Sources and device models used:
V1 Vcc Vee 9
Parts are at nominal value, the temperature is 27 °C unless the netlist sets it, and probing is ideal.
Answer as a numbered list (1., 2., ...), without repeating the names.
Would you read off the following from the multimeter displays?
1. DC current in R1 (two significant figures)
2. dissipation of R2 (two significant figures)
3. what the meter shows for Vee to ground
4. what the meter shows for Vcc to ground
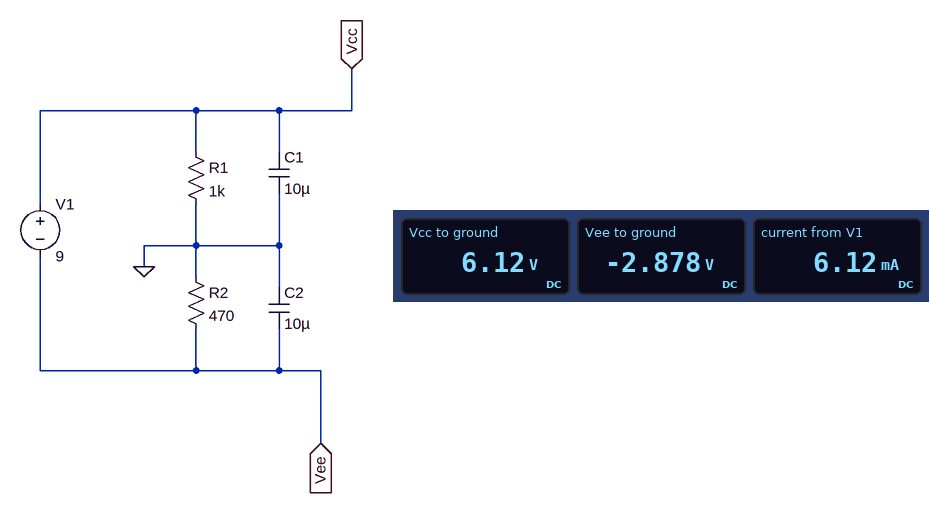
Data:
1. 6.1 mA
2. 18 mW
3. -2.878 V
4. 6.12 V
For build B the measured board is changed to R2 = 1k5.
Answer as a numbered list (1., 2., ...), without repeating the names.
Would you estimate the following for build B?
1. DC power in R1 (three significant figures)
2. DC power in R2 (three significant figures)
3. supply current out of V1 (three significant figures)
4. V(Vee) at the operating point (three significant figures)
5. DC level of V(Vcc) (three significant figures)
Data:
1. 13.0 mW
2. 19.4 mW
3. 3.60 mA
4. -5.40 V
5. 3.60 V
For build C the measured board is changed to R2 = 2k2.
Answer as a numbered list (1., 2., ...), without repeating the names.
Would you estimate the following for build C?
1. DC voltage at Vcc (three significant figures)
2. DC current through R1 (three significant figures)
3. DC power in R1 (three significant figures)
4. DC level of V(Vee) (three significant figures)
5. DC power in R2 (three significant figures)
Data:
1. 2.81 V
2. 2.81 mA
3. 7.91 mW
4. -6.19 V
5. 17.4 mW
